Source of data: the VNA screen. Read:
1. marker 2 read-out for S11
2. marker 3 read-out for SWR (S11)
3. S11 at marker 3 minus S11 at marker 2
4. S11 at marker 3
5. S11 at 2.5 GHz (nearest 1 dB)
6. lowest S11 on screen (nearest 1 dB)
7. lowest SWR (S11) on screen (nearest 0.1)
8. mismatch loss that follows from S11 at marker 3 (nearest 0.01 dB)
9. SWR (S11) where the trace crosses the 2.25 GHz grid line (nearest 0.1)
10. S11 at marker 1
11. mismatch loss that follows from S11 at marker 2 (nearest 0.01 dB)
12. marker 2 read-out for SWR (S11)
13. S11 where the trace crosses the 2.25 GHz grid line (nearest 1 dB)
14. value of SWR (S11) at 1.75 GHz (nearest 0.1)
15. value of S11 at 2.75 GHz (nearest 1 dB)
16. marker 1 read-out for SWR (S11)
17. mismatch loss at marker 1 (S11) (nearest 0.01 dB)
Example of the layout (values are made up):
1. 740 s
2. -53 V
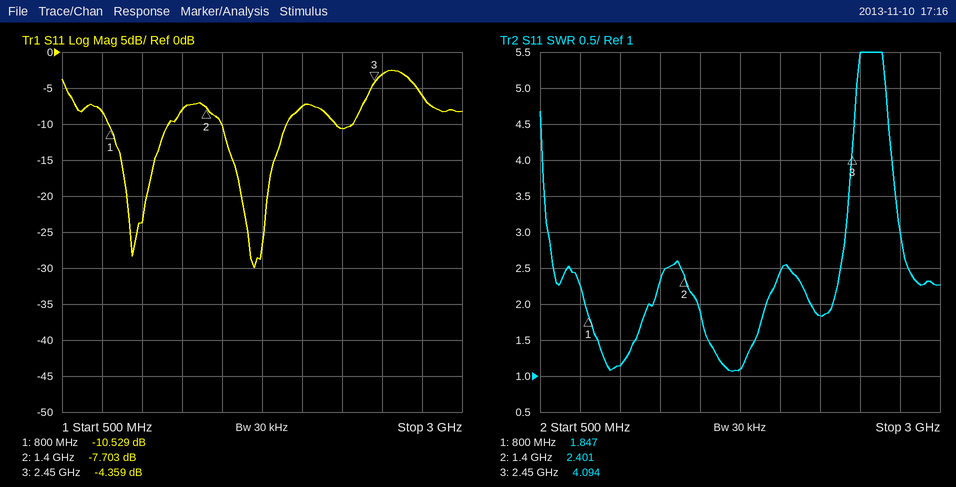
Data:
1. -7.703 dB
2. 4.094
3. 3.344 dB
4. -4.359 dB
5. -3 dB
6. -30 dB
7. 1.1
8. 1.98 dB
9. 1.8
10. -10.529 dB
11. 0.81 dB
12. 2.401
13. -11 dB
14. 1.1
15. -6 dB
16. 1.847
17. 0.40 dB
